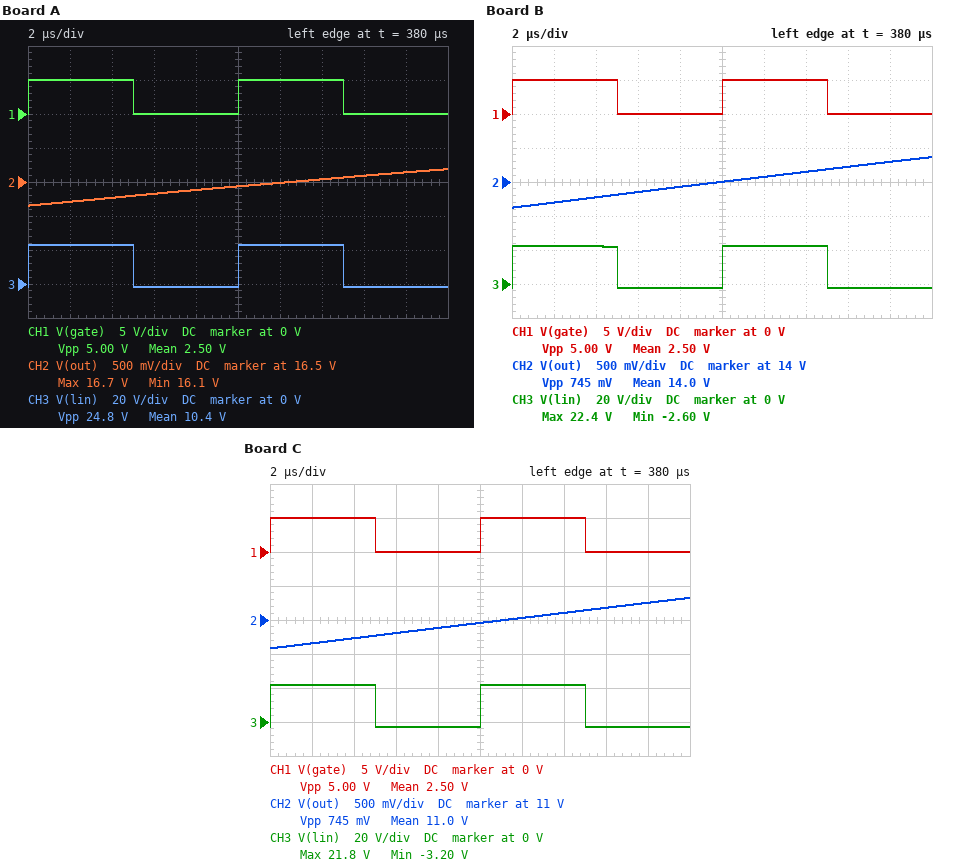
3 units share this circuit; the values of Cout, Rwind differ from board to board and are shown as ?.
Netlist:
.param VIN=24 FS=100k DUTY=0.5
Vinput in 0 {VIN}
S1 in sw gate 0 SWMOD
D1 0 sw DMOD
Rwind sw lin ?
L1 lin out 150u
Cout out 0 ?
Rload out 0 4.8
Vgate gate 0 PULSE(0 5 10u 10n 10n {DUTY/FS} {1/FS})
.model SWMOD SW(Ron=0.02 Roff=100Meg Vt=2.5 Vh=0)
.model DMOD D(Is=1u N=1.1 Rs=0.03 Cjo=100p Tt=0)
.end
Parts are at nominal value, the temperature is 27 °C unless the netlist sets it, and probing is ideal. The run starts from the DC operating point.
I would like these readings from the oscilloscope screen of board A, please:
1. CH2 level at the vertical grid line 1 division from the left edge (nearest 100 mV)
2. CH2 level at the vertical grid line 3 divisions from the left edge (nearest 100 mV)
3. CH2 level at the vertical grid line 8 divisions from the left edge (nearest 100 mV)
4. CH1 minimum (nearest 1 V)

16.2 V
16.3 V
16.6 V
0 V
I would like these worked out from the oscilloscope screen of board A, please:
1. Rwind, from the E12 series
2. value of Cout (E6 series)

0.15 Ω
150 µF
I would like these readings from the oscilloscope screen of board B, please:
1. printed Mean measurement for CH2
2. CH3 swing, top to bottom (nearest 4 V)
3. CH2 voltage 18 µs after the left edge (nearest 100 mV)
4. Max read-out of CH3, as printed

14.0 V
24 V
14.3 V
22.4 V
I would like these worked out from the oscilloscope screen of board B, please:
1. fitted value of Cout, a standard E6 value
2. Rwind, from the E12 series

220 µF
0.15 Ω
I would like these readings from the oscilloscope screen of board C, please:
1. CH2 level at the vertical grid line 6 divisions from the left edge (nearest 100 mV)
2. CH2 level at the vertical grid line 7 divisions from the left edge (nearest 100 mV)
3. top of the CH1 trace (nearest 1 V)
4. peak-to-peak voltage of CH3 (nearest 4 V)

11.0 V
11.1 V
5 V
24 V
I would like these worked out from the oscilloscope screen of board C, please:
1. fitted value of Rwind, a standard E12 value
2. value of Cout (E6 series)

0.15 Ω
330 µF
